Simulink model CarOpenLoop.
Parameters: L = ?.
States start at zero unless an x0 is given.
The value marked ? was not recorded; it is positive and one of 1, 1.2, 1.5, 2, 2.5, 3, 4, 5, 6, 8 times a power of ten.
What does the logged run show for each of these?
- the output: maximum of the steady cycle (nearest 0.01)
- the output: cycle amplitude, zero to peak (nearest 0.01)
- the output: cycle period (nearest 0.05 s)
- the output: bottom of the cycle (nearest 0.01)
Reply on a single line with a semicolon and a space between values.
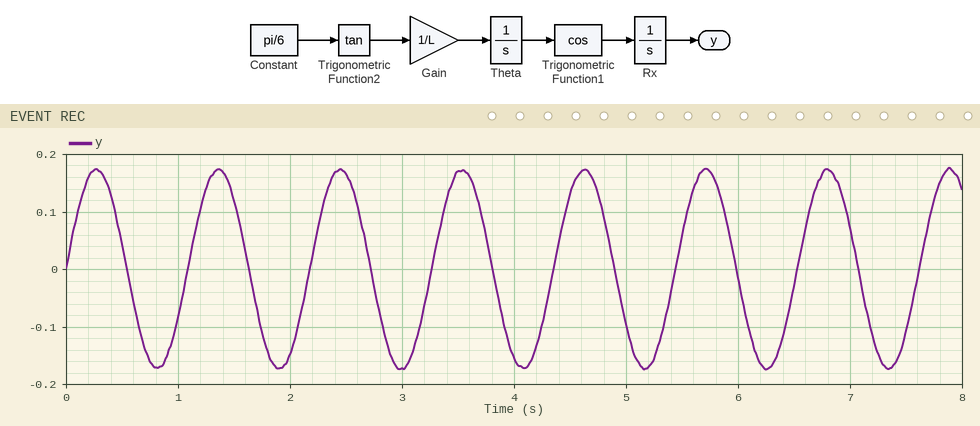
0.17; 0.17; 1.10 s; -0.17
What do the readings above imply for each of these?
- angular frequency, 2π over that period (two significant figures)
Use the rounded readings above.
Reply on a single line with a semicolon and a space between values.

5.7 rad/s
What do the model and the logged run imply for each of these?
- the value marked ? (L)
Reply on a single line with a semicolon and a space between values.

0.1
